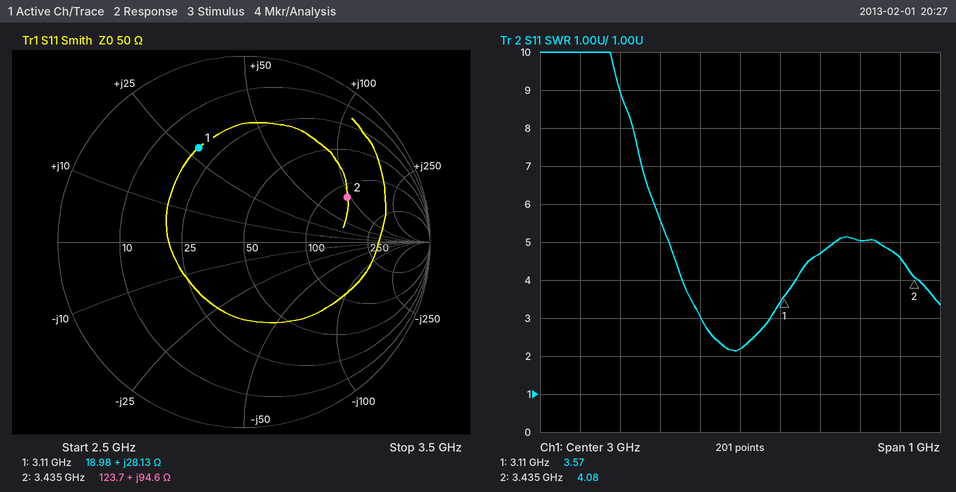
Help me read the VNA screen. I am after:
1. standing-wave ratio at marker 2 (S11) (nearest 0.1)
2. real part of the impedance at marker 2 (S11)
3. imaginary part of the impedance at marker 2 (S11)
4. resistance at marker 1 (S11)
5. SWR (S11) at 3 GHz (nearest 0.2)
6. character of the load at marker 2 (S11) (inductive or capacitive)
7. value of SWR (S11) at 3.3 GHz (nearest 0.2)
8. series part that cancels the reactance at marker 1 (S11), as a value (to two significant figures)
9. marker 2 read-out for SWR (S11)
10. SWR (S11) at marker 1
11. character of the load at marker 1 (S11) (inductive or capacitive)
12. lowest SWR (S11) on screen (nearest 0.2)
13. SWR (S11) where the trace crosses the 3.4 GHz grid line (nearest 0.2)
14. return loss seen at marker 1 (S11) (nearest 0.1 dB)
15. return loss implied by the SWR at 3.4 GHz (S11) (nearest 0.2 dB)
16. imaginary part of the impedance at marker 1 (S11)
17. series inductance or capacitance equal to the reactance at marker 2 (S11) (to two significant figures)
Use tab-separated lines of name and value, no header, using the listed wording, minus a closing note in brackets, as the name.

standing-wave ratio at marker 2 (S11)	4.1
real part of the impedance at marker 2	123.7 Ω
imaginary part of the impedance at marker 2	+94.6 Ω
resistance at marker 1	18.98 Ω
SWR (S11) at 3 GHz	2.2
character of the load at marker 2 (S11)	inductive
value of SWR (S11) at 3.3 GHz	5.0
series part that cancels the reactance at marker 1 (S11), as a value	1.8 pF
marker 2 read-out for SWR	4.08
SWR (S11) at marker 1	3.57
character of the load at marker 1 (S11)	inductive
lowest SWR (S11) on screen	2.2
SWR (S11) where the trace crosses the 3.4 GHz grid line	4.6
return loss seen at marker 1 (S11)	5.0 dB
return loss implied by the SWR at 3.4 GHz (S11)	3.8 dB
imaginary part of the impedance at marker 1	+28.13 Ω
series inductance or capacitance equal to the reactance at marker 2 (S11)	4.4 nH
